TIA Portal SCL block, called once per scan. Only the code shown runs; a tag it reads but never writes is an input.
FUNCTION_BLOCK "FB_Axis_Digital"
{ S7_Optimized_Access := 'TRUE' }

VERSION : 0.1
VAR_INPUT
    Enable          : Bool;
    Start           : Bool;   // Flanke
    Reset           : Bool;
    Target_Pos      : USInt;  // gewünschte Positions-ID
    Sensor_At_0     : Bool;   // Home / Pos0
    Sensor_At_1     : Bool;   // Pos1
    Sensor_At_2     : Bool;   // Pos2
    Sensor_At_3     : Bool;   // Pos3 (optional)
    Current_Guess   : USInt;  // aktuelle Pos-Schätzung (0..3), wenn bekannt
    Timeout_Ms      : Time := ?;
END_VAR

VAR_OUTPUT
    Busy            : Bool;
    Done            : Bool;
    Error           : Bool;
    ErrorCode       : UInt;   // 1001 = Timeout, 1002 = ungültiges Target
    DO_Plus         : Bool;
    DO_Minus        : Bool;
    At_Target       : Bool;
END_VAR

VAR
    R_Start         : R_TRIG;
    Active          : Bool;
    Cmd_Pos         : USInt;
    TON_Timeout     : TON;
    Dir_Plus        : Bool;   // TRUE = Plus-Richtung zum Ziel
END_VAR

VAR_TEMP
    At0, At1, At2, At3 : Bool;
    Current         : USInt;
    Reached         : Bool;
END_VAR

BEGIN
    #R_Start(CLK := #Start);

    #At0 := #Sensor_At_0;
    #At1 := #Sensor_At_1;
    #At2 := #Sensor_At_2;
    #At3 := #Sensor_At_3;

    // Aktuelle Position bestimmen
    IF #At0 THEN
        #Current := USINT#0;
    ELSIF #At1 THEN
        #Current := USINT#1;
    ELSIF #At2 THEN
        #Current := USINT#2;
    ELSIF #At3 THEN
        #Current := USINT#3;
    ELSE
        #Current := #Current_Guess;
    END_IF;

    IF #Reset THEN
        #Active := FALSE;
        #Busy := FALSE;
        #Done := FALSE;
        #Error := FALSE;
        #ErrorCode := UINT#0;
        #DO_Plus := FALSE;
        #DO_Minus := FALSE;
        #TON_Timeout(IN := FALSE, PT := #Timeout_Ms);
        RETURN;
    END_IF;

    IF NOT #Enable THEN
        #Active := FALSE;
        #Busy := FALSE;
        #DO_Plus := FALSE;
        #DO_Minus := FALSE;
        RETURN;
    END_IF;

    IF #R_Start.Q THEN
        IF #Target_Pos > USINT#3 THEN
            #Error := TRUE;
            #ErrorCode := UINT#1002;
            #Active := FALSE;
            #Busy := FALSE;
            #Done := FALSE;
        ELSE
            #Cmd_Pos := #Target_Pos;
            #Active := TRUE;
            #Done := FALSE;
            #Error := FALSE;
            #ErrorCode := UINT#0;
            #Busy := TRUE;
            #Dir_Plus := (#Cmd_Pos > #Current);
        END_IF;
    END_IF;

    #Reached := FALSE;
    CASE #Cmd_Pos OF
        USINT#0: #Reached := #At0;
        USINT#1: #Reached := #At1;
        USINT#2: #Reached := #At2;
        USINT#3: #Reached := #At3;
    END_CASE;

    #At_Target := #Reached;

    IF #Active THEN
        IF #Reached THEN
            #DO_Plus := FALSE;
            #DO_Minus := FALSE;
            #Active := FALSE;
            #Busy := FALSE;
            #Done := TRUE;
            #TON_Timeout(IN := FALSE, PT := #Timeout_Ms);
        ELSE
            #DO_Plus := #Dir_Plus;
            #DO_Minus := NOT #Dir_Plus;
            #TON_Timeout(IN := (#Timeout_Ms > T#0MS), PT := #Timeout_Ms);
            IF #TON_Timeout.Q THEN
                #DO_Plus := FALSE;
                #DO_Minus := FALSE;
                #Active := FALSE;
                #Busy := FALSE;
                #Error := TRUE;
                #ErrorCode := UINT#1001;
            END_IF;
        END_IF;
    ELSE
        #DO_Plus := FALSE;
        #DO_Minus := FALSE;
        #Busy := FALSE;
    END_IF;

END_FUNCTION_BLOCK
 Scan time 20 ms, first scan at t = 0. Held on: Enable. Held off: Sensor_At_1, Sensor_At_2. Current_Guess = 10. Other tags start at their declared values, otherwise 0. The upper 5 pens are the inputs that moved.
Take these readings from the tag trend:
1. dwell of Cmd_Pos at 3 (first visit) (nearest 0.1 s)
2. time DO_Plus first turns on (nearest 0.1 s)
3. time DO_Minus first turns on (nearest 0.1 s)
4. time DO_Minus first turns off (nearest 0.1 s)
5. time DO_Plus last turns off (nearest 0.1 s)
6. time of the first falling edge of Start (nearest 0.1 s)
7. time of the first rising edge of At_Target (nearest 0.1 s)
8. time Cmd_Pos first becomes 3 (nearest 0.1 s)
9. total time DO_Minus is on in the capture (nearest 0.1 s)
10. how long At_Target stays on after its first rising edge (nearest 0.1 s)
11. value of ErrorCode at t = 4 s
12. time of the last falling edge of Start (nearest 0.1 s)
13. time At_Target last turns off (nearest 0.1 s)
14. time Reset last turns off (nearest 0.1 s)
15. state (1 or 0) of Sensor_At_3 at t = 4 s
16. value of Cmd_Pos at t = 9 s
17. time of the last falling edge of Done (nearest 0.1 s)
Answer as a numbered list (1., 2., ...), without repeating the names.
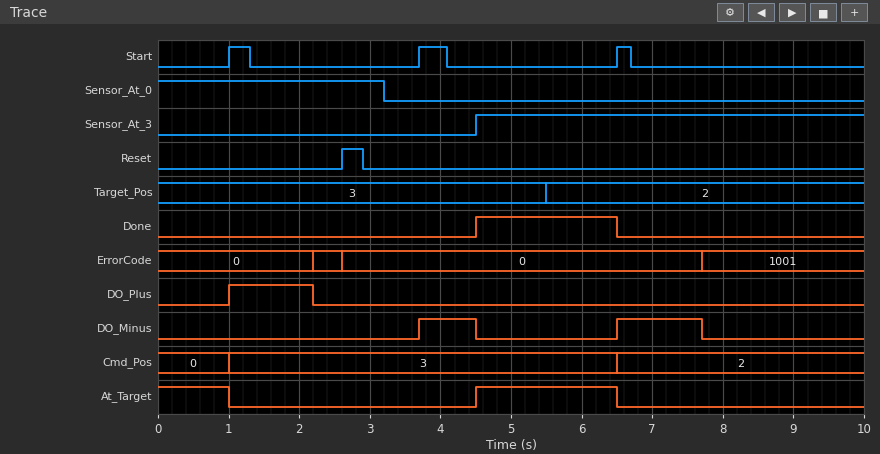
1. 5.5 s
2. 1.0 s
3. 3.7 s
4. 4.5 s
5. 2.2 s
6. 1.3 s
7. 4.5 s
8. 1.0 s
9. 2.0 s
10. 2.0 s
11. 0
12. 6.7 s
13. 6.5 s
14. 2.9 s
15. 0
16. 2
17. 6.5 s
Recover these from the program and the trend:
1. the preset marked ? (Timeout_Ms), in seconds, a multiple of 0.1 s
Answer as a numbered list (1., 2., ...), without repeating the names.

1. 1.2 s
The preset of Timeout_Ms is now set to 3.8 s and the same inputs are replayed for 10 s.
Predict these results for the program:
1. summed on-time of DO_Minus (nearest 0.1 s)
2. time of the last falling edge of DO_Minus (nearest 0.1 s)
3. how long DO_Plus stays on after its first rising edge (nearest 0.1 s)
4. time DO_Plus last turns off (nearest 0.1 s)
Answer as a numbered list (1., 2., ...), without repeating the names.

1. 4.3 s
2. 4.5 s
3. 1.6 s
4. 2.6 s
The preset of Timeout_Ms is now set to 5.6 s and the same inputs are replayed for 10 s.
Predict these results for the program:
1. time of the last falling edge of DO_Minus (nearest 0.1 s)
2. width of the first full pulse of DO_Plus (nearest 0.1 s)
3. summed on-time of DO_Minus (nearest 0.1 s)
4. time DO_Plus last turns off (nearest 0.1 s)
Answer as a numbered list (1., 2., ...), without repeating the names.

1. 4.5 s
2. 1.6 s
3. 4.3 s
4. 2.6 s
